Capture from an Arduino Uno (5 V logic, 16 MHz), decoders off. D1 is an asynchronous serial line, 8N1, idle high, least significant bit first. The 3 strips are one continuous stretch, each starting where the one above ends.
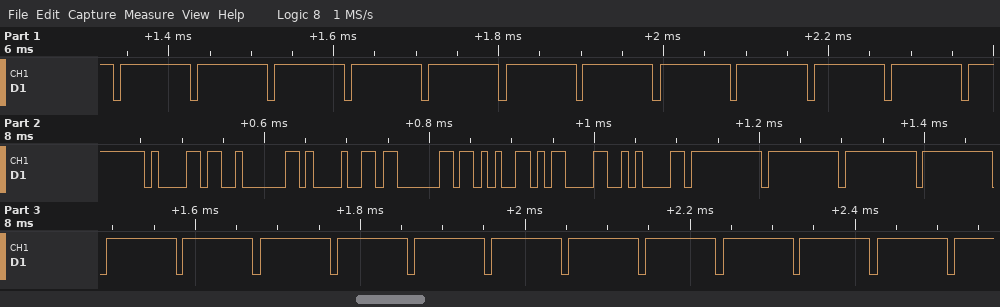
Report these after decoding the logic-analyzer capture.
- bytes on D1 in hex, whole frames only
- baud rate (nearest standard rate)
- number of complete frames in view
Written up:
0xFF 0xFF 0xFF 0xFF 0xFF 0xFF 0xFF 0xFF 0xFF 0xFF 0xFF 0xFF 0x61 0x02 0x21 0x03 0x2B 0x0D 0x0A 0xFF 0xFF 0xFF 0xFF 0xFF 0xFF 0xFF 0xFF 0xFF 0xFF 0xFF 0xFF 0xFF 0xFF 0xFF
115200 baud
34
